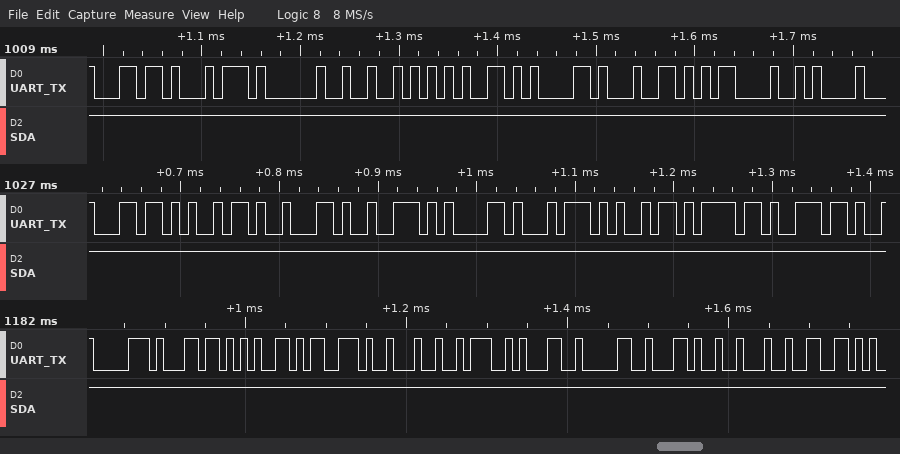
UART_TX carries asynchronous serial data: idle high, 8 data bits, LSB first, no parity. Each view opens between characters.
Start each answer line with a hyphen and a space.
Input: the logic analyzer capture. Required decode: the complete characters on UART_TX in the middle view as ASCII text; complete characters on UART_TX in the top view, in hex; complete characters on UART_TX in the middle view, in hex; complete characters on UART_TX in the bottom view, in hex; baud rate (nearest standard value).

- "libration"
- 6C, 74, 20, 52, 65, 61, 64, 0D, 0A
- 6C, 69, 62, 72, 61, 74, 69, 6F, 6E
- 70, 6C, 65, 73, 22, 3A, 31, 30, 2C, 22, 66
- 115200 baud
